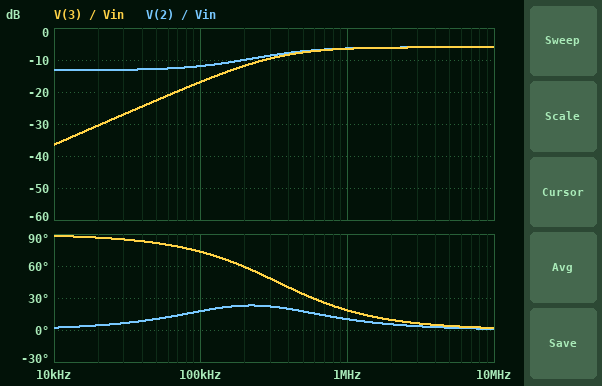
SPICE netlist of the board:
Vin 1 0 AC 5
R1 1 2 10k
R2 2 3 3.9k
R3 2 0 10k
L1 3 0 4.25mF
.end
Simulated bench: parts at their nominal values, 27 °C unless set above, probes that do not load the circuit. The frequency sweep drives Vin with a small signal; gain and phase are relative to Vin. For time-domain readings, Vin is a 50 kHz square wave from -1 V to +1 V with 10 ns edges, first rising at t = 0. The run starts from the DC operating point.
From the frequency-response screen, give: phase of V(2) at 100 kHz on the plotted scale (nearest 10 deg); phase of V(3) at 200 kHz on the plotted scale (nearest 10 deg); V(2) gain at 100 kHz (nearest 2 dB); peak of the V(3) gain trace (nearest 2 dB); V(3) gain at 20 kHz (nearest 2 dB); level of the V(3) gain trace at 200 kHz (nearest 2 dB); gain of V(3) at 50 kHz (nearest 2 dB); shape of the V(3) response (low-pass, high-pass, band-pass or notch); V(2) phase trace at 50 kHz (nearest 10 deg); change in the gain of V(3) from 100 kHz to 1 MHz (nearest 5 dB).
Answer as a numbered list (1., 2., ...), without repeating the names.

1. 20 deg
2. 60 deg
3. -12 dB
4. -6 dB
5. -30 dB
6. -12 dB
7. -22 dB
8. high-pass
9. 10 deg
10. 10 dB
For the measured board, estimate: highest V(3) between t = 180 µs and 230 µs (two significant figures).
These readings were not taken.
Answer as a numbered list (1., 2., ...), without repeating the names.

1. 990 mV
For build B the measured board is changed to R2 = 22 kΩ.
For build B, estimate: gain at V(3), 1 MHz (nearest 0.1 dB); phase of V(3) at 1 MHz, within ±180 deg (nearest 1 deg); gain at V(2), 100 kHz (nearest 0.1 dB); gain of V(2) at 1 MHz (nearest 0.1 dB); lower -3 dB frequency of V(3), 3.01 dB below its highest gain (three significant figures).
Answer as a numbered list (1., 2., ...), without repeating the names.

1. -9.1 dB
2. 45 deg
3. -7.8 dB
4. -6.8 dB
5. 1.01 MHz
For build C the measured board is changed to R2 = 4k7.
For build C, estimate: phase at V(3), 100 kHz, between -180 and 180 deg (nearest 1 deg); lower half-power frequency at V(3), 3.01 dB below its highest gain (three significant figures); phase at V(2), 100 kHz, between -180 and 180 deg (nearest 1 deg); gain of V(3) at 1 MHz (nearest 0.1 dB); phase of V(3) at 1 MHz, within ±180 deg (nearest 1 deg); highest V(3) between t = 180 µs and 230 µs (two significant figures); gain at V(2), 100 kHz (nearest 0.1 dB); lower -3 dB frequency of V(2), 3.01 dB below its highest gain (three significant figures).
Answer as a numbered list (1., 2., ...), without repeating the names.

1. 75 deg
2. 363 kHz
3. 14 deg
4. -6.6 dB
5. 20 deg
6. 990 mV
7. -11.4 dB
8. 265 kHz
